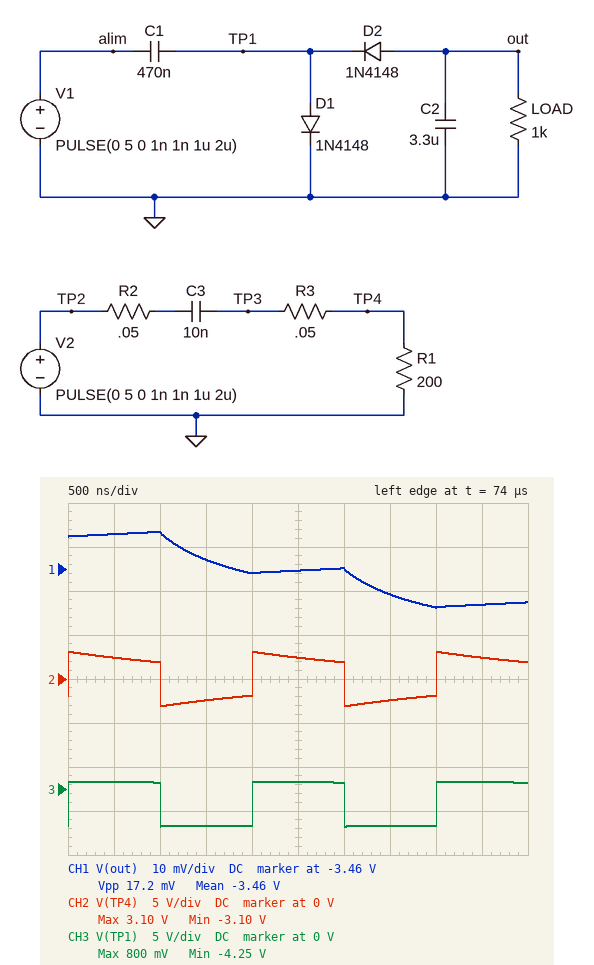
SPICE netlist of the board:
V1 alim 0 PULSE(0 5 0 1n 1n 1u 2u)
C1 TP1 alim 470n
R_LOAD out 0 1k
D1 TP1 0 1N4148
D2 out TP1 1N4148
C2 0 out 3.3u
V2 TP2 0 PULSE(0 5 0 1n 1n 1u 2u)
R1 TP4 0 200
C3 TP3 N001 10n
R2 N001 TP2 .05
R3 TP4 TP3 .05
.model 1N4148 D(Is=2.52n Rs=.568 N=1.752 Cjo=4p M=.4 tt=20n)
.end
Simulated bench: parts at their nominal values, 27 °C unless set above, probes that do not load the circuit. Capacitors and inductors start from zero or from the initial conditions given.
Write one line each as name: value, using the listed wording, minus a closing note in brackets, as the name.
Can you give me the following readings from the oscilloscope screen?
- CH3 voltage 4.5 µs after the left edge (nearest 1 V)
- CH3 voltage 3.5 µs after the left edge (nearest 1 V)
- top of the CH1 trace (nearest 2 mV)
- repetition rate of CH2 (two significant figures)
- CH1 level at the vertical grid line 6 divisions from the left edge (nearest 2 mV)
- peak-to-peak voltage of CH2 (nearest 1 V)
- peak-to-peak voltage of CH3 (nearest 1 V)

CH3 voltage 4.5 µs after the left edge: 1 V
CH3 voltage 3.5 µs after the left edge: -4 V
top of the CH1 trace: -3.452 V
repetition rate of CH2: 500 kHz
CH1 level at the vertical grid line 6 divisions from the left edge: -3.460 V
peak-to-peak voltage of CH2: 6 V
peak-to-peak voltage of CH3: 5 V
